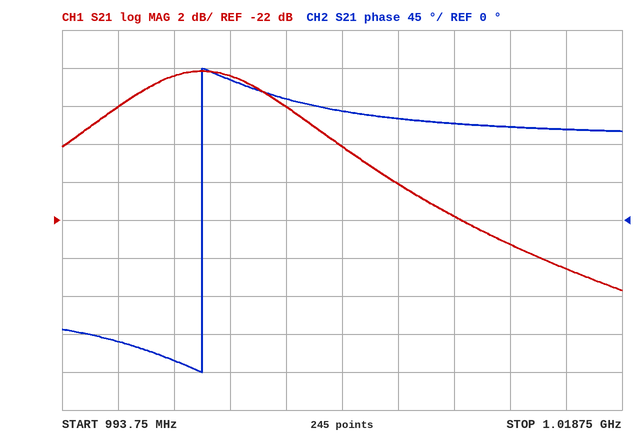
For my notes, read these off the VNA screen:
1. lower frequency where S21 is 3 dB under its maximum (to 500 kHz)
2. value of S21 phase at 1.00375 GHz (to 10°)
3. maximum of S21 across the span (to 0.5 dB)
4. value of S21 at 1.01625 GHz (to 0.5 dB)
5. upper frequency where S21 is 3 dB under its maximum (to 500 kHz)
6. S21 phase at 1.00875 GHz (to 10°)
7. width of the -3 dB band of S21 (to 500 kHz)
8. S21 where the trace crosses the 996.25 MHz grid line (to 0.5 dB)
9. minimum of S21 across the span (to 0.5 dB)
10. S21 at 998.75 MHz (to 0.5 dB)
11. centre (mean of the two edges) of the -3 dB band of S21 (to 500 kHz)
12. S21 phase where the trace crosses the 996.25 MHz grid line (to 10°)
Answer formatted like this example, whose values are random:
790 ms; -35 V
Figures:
995.0 MHz; 140°; -14.0 dB; -24.5 dB; 1.0050 GHz; 120°; 10.0 MHz; -16.0 dB; -25.5 dB; -14.5 dB; 1.0000 GHz; -140°
